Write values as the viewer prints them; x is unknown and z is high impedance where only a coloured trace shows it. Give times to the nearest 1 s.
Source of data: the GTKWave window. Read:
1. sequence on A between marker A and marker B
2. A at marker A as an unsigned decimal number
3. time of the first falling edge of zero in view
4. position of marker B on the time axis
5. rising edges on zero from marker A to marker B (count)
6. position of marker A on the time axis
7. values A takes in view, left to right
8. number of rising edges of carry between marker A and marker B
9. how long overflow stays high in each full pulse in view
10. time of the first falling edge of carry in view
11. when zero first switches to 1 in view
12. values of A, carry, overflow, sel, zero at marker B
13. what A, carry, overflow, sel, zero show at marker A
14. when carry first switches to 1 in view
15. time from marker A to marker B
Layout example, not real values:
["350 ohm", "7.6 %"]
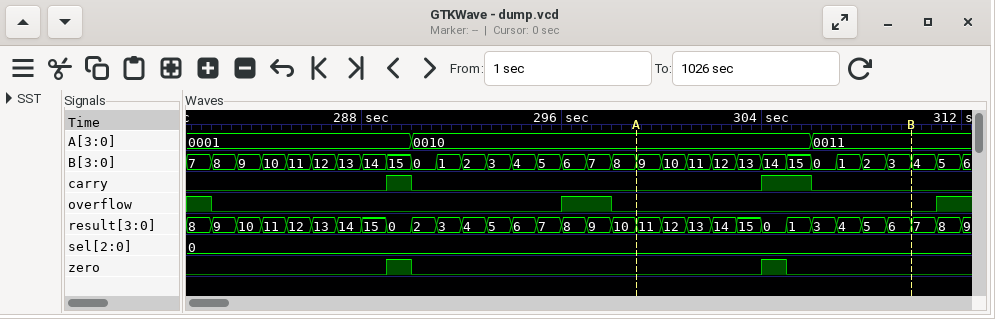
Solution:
["0010, 0011", "2", "290 s", "310 s", "1", "299 s", "0001, 0010, 0011", "1", "2 s", "290 s", "289 s", "A=0011, carry=0, overflow=0, sel=0, zero=0", "A=0010, carry=0, overflow=0, sel=0, zero=0", "289 s", "11 s"]
